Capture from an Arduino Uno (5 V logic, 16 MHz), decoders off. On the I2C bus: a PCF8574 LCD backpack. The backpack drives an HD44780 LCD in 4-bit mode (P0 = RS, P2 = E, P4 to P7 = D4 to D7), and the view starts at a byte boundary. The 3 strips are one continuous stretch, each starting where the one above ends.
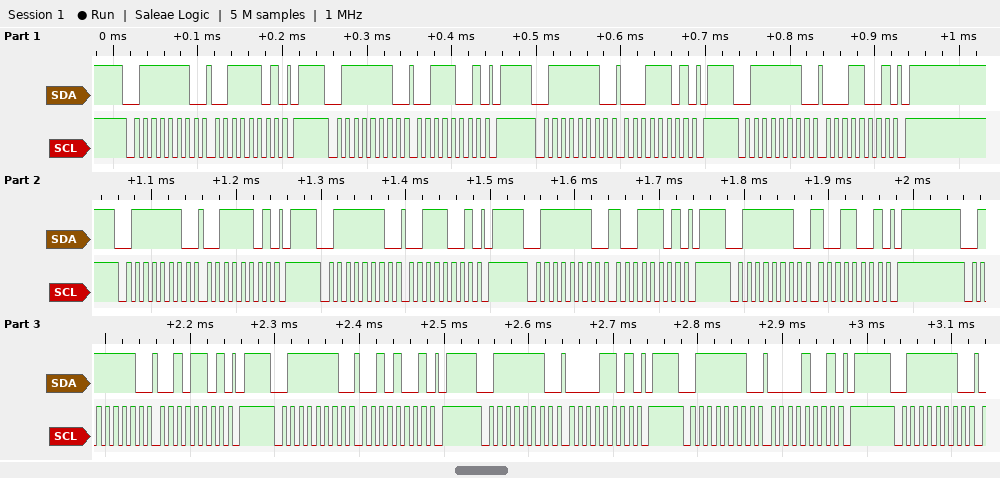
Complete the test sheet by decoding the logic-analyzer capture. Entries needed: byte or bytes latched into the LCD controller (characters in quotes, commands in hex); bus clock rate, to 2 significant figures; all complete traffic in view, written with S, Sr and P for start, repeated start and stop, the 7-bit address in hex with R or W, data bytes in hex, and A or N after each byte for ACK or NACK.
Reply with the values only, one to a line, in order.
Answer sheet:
'1' '9' ' '
100 kHz
S 3FW A 3D A P S 3FW A 39 A P S 3FW A 1D A P S 3FW A 19 A P S 3FW A 3D A P S 3FW A 39 A P S 3FW A 9D A P S 3FW A 99 A P S 3FW A 2D A P S 3FW A 29 A P S 3FW A 0D A P S 3FW A 09 A P S 3FW A
